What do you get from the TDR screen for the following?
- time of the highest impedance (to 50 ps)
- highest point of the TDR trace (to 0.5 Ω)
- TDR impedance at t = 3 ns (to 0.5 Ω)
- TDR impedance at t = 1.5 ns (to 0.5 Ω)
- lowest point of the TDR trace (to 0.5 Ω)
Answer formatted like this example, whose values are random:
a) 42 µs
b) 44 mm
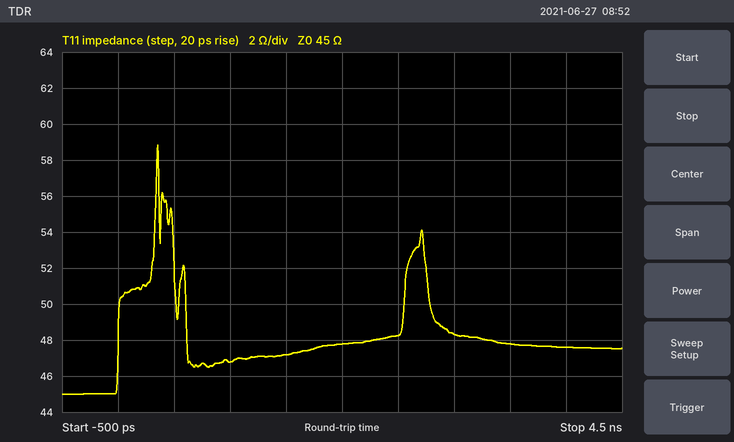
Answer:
a) 350 ps
b) 59.0 Ω
c) 48.5 Ω
d) 47.0 Ω
e) 45.0 Ω
